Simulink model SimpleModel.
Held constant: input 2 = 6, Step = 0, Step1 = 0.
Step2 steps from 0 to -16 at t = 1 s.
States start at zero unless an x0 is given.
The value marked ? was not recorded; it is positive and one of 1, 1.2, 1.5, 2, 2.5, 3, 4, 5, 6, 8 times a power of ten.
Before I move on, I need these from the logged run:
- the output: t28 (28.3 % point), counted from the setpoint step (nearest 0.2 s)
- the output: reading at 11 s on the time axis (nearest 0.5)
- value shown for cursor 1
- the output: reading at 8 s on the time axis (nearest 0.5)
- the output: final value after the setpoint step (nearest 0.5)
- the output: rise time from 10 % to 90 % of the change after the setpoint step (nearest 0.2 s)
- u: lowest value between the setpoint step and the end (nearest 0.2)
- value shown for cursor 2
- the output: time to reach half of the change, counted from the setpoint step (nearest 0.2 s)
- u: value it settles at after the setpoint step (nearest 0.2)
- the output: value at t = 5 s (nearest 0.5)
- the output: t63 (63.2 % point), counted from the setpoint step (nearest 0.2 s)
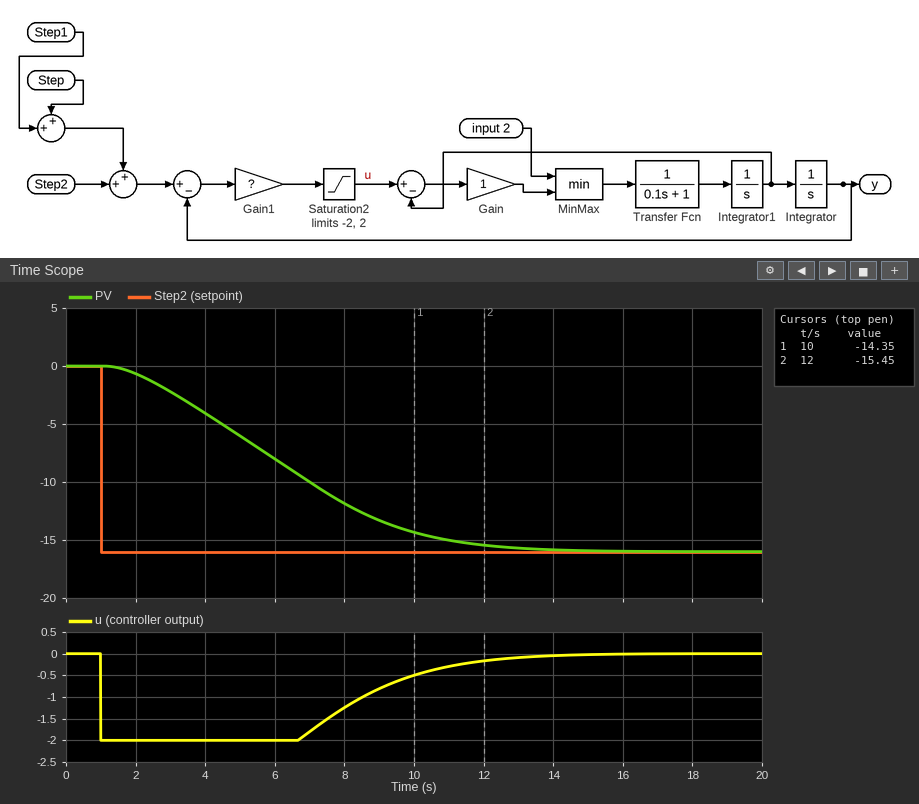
3.2 s
-15.0
-14.35
-12.0
-16.0
7.4 s
-2.0
-15.45
5.0 s
0.0
-6.0
6.0 s
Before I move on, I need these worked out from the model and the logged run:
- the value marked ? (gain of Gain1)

0.3
